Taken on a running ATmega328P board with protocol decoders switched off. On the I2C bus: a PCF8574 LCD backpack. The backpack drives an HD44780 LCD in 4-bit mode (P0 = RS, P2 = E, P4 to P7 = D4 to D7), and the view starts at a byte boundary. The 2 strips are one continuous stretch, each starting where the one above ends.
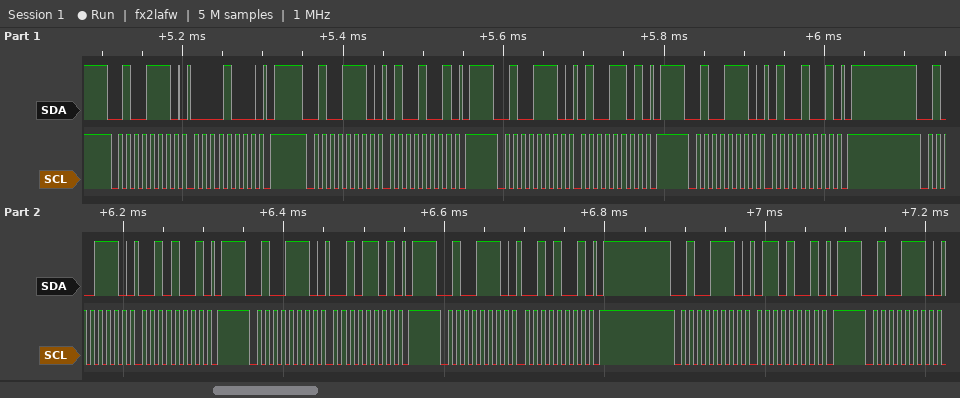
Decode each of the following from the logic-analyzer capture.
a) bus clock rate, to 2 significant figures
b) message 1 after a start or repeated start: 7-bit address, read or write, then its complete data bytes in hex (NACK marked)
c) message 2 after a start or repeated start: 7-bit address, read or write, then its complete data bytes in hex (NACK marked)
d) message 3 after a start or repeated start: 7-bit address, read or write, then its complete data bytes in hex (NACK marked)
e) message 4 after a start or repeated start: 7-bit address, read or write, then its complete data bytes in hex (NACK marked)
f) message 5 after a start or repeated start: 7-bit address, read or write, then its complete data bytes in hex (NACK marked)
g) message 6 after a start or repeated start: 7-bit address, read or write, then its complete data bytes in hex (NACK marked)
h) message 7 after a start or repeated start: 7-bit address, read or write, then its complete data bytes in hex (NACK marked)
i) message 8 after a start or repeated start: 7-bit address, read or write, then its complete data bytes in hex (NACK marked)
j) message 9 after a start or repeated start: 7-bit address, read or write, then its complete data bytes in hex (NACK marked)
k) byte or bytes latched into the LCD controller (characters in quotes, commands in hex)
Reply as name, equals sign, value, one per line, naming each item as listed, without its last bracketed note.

bus clock rate, to 2 significant figures = 100 kHz
message 1 after a start or repeated start: 7-bit address, read or write, then its complete data bytes in hex = 0x27 write: 08
message 2 after a start or repeated start: 7-bit address, read or write, then its complete data bytes in hex = 0x27 write: 49
message 3 after a start or repeated start: 7-bit address, read or write, then its complete data bytes in hex = 0x27 write: 4D
message 4 after a start or repeated start: 7-bit address, read or write, then its complete data bytes in hex = 0x27 write: 49
message 5 after a start or repeated start: 7-bit address, read or write, then its complete data bytes in hex = 0x27 write: 29
message 6 after a start or repeated start: 7-bit address, read or write, then its complete data bytes in hex = 0x27 write: 2D
message 7 after a start or repeated start: 7-bit address, read or write, then its complete data bytes in hex = 0x27 write: 29
message 8 after a start or repeated start: 7-bit address, read or write, then its complete data bytes in hex = 0x27 write: 69
message 9 after a start or repeated start: 7-bit address, read or write, then its complete data bytes in hex = 0x27 write
byte or bytes latched into the LCD controller = 'B'
